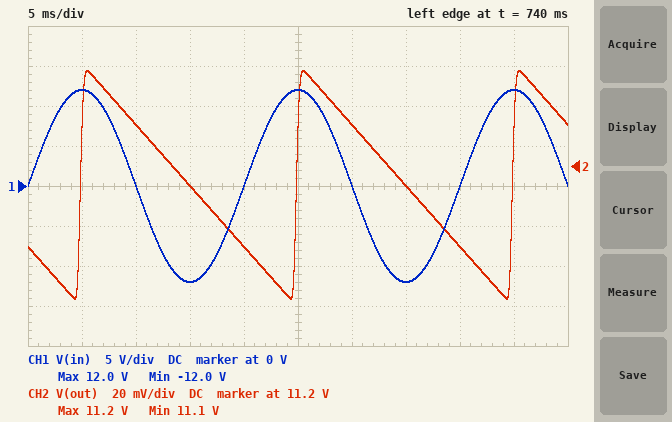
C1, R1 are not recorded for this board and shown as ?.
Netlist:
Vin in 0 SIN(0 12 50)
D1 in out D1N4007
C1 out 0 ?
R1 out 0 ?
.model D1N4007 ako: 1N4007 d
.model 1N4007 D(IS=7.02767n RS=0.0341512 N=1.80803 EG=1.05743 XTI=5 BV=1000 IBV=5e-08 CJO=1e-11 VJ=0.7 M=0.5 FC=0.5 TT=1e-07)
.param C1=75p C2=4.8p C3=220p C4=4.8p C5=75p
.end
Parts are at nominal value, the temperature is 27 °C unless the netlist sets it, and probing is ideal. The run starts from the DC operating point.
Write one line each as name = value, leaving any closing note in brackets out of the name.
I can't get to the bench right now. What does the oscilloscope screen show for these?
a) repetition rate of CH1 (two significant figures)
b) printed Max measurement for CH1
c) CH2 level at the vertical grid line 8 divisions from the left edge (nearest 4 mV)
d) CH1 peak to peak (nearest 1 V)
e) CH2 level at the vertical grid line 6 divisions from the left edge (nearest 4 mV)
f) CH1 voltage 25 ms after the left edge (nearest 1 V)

repetition rate of CH1 = 50 Hz
printed Max measurement for CH1 = 12.0 V
CH2 level at the vertical grid line 8 divisions from the left edge = 11.160 V
CH1 peak to peak = 24 V
CH2 level at the vertical grid line 6 divisions from the left edge = 11.220 V
CH1 voltage 25 ms after the left edge = 12 V
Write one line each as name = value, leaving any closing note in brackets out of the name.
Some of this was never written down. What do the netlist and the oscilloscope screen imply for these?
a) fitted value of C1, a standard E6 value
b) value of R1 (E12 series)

fitted value of C1, a standard E6 value = 680 µF
value of R1 = 2.7 kΩ
